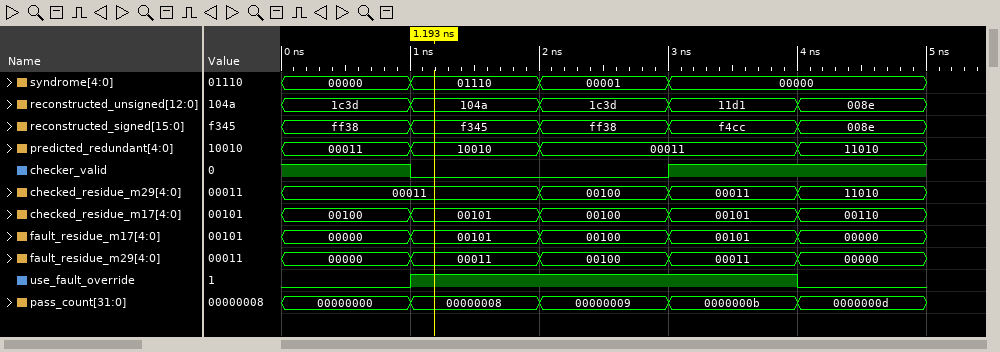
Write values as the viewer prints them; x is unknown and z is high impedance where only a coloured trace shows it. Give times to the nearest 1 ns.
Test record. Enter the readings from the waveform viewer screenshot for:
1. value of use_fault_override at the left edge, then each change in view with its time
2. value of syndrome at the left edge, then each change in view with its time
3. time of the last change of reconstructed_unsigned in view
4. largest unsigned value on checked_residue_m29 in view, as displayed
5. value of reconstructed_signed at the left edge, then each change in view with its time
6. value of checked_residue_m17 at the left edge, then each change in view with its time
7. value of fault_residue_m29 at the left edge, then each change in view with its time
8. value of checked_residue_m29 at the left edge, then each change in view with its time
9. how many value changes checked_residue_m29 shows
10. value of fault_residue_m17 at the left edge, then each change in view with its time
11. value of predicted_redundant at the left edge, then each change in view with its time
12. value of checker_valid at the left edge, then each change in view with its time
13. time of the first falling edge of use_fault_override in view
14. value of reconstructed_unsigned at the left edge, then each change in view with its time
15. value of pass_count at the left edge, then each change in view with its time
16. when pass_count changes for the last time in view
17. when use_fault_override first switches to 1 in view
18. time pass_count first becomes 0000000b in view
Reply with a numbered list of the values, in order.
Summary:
1. 0, 1 at 1 ns, 0 at 4 ns
2. 00000, 01110 at 1 ns, 00001 at 2 ns, 00000 at 3 ns
3. 4 ns
4. 11010
5. ff38, f345 at 1 ns, ff38 at 2 ns, f4cc at 3 ns, 008e at 4 ns
6. 00100, 00101 at 1 ns, 00100 at 2 ns, 00101 at 3 ns, 00110 at 4 ns
7. 00000, 00011 at 1 ns, 00100 at 2 ns, 00011 at 3 ns, 00000 at 4 ns
8. 00011, 00100 at 2 ns, 00011 at 3 ns, 11010 at 4 ns
9. 3
10. 00000, 00101 at 1 ns, 00100 at 2 ns, 00101 at 3 ns, 00000 at 4 ns
11. 00011, 10010 at 1 ns, 00011 at 2 ns, 11010 at 4 ns
12. 1, 0 at 1 ns, 1 at 3 ns
13. 4 ns
14. 1c3d, 104a at 1 ns, 1c3d at 2 ns, 11d1 at 3 ns, 008e at 4 ns
15. 00000000, 00000008 at 1 ns, 00000009 at 2 ns, 0000000b at 3 ns, 0000000d at 4 ns
16. 4 ns
17. 1 ns
18. 3 ns
